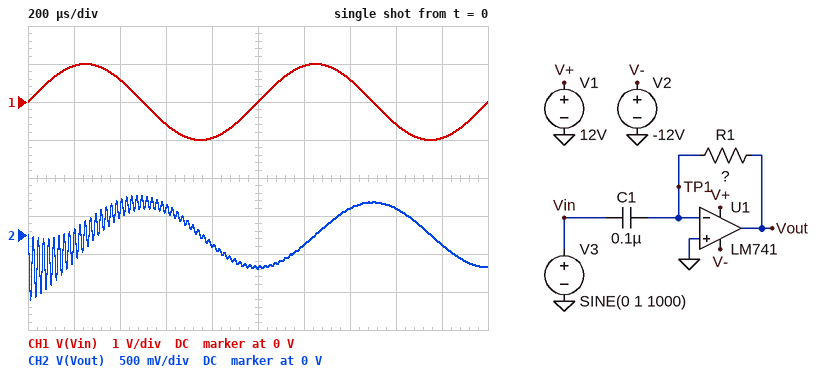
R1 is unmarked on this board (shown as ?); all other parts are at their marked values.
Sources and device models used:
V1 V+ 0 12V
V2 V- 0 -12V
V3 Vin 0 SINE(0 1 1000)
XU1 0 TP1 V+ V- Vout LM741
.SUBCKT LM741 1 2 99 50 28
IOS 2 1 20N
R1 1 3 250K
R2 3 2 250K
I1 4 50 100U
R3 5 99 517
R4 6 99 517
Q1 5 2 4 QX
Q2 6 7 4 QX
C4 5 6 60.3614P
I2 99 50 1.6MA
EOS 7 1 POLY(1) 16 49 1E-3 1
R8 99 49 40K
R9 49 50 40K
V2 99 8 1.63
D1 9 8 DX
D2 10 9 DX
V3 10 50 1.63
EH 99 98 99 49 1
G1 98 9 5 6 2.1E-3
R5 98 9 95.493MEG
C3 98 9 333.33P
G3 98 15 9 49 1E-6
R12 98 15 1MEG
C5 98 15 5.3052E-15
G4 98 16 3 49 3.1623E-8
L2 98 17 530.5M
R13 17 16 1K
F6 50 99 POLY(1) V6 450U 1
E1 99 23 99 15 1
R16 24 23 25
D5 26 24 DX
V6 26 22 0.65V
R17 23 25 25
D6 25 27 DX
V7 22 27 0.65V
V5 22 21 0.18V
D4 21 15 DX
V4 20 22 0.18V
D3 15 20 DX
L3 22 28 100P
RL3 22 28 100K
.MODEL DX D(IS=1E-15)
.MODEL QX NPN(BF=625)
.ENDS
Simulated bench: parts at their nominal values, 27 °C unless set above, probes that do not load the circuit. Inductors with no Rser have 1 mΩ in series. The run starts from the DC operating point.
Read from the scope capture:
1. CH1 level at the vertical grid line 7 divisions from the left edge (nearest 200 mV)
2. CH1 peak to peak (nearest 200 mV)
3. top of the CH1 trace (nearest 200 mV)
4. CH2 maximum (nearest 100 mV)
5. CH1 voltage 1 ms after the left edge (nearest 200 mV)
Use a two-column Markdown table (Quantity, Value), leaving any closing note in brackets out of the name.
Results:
| Quantity | Value |
|---|---|
| CH1 level at the vertical grid line 7 divisions from the left edge | 600 mV |
| CH1 peak to peak | 2.0 V |
| top of the CH1 trace | 1.0 V |
| CH2 maximum | 500 mV |
| CH1 voltage 1 ms after the left edge | 0 V |
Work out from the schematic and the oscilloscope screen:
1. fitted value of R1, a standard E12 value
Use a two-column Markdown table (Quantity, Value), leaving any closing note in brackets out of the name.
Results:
| Quantity | Value |
|---|---|
| fitted value of R1, a standard E12 value | 680 Ω |
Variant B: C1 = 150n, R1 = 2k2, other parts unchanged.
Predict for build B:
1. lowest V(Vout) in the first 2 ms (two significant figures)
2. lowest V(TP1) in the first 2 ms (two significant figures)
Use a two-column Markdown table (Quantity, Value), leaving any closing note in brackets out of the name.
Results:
| Quantity | Value |
|---|---|
| lowest V(Vout) in the first 2 ms | -4.1 V |
| lowest V(TP1) in the first 2 ms | -48 mV |
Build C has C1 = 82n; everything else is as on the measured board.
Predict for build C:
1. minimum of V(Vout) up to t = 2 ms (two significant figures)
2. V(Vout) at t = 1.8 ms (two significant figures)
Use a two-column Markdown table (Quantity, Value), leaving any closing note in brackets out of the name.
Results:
| Quantity | Value |
|---|---|
| minimum of V(Vout) up to t = 2 ms | -700 mV |
| V(Vout) at t = 1.8 ms | -110 mV |
